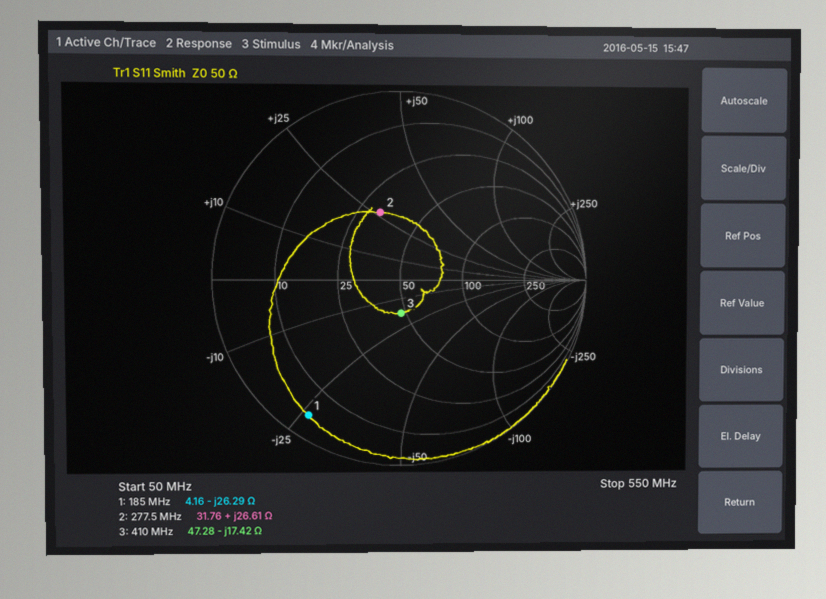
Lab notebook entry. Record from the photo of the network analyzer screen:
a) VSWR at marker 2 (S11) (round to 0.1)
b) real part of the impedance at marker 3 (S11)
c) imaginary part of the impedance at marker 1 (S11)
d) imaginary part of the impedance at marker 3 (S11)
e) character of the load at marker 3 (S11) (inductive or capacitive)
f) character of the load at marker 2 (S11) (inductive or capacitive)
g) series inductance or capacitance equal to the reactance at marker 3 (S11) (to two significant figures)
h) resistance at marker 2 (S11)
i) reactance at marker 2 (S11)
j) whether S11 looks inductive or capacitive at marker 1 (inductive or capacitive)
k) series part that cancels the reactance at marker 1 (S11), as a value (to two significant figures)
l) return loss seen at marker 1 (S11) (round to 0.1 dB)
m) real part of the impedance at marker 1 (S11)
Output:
2.2
47.28 Ω
-26.29 Ω
-17.42 Ω
capacitive
inductive
22 pF
31.76 Ω
+26.61 Ω
capacitive
23 nH
1.1 dB
4.16 Ω
